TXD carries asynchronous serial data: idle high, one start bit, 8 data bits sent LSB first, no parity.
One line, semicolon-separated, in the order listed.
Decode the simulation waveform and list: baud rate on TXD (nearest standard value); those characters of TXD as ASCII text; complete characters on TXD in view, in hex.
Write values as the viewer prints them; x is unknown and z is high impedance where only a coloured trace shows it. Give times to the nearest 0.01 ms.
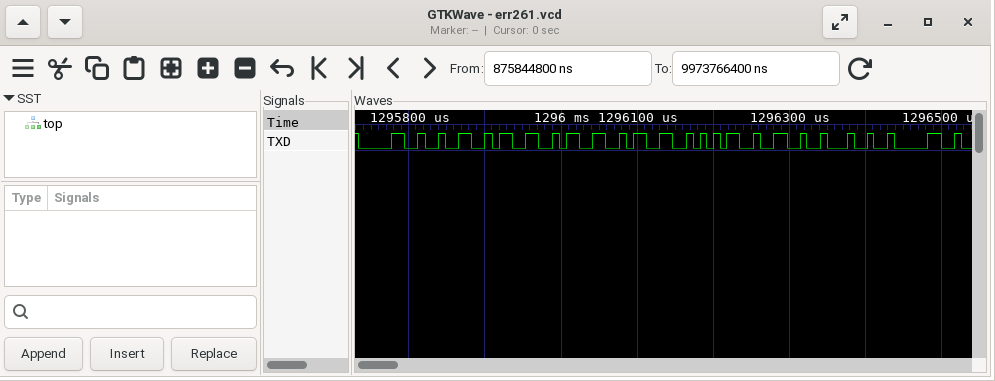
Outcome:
115200 baud; "023335&$0"; 30, 32, 33, 33, 33, 35, 26, 24, 30
